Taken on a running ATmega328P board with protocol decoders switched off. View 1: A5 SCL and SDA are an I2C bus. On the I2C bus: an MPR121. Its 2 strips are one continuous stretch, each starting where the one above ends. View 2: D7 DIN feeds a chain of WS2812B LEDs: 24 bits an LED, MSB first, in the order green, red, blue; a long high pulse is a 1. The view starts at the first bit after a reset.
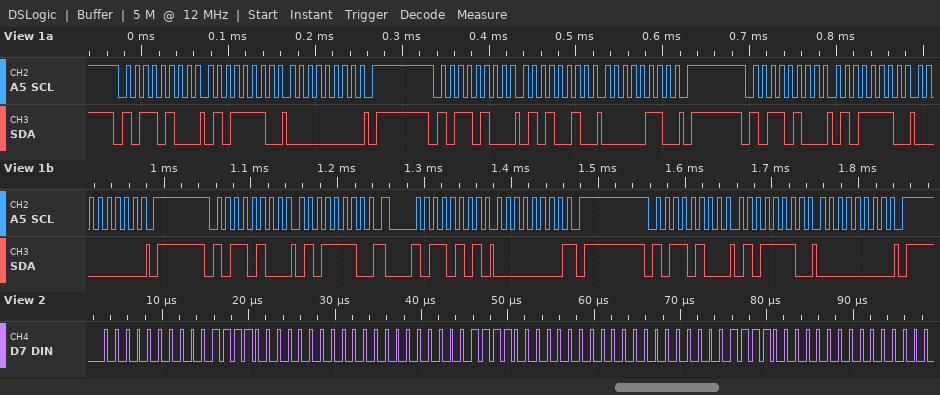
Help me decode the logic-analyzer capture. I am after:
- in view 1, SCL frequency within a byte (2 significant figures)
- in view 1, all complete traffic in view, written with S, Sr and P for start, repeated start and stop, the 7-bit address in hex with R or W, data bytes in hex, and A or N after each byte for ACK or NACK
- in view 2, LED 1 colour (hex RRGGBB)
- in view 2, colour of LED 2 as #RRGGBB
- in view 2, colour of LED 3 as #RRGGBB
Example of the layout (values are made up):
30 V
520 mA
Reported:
100 kHz
S 5AW A 5E A 00 A P S 5AW A 52 A 06 A P S 5AW A 5E A 00 A P S 5AW A 5E A Sr 5AR A 00 N P S 5AW A 5E A 00 A P
#3C0000
#3C0000
#3C0000
